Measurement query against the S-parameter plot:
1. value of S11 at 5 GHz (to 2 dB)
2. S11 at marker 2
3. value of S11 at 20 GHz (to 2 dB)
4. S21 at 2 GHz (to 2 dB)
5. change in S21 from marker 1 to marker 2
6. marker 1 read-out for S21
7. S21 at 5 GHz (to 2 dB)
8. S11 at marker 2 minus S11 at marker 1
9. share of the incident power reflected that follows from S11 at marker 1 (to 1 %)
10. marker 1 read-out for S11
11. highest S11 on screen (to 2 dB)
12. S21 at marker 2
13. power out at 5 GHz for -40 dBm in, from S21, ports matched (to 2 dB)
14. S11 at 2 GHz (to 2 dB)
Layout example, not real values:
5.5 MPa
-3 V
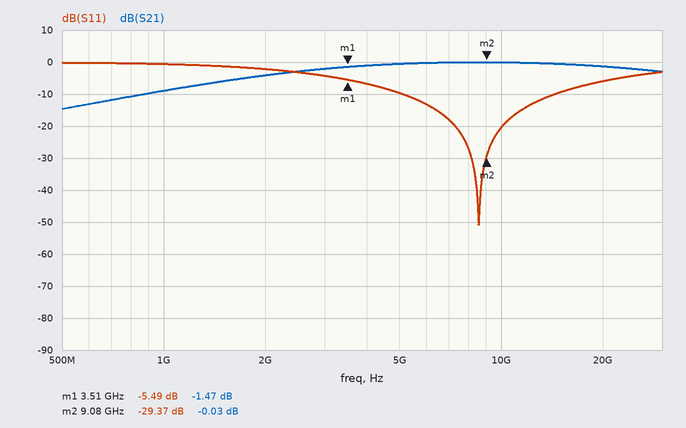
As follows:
-10 dB
-29.37 dB
-6 dB
-4 dB
1.44 dB
-1.47 dB
0 dB
-23.88 dB
28 %
-5.49 dB
0 dB
-0.03 dB
-40 dBm
-2 dB
